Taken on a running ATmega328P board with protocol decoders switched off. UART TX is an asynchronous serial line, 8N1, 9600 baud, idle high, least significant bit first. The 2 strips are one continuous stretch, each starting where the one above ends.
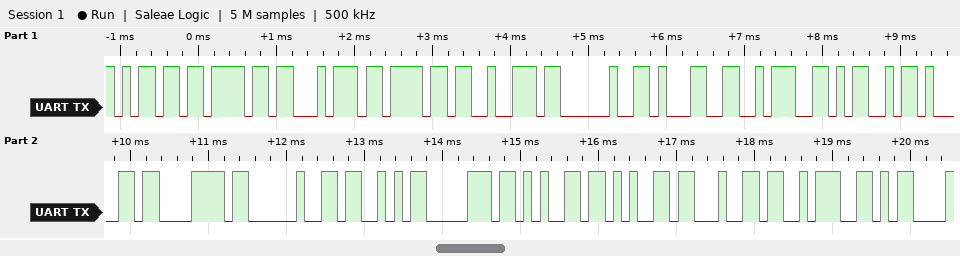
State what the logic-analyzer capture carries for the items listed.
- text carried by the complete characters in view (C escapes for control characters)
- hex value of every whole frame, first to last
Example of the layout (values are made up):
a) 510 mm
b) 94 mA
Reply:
a) "motor 1:Max Speed:\r"
b) 6D 6F 74 6F 72 20 31 3A 4D 61 78 20 53 70 65 65 64 3A 0D
